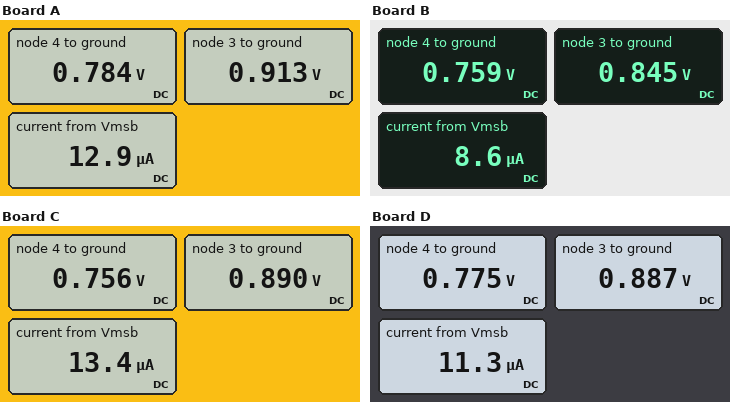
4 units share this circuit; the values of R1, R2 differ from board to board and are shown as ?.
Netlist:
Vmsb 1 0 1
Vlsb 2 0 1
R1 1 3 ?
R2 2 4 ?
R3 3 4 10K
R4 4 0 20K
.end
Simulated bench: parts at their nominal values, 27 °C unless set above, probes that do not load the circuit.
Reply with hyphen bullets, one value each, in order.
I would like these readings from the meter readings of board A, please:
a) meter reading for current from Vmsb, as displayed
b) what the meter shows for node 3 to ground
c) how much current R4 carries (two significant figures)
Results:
- 12.9 µA
- 0.913 V
- 39 µA
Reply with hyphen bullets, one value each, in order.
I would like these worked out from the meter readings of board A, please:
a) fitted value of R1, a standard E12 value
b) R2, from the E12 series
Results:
- 6.8 kΩ
- 8.2 kΩ
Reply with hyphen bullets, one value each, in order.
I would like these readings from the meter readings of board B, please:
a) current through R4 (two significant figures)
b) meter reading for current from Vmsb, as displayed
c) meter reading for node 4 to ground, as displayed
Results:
- 38 µA
- 8.6 µA
- 0.759 V
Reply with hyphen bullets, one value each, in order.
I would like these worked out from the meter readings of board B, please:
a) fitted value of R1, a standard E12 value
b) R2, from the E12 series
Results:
- 18 kΩ
- 8.2 kΩ
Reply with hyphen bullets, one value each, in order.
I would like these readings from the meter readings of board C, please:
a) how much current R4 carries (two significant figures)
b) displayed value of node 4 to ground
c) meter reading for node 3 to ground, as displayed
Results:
- 38 µA
- 0.756 V
- 0.890 V
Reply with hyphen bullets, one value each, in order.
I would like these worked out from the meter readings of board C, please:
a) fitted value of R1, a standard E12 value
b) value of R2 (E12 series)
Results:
- 8.2 kΩ
- 10 kΩ
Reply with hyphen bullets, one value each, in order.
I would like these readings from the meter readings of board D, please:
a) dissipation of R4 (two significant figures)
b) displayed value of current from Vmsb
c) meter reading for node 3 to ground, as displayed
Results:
- 30 µW
- 11.3 µA
- 0.887 V
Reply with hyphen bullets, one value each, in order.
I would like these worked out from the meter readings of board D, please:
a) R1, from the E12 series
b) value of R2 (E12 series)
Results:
- 10 kΩ
- 8.2 kΩ
